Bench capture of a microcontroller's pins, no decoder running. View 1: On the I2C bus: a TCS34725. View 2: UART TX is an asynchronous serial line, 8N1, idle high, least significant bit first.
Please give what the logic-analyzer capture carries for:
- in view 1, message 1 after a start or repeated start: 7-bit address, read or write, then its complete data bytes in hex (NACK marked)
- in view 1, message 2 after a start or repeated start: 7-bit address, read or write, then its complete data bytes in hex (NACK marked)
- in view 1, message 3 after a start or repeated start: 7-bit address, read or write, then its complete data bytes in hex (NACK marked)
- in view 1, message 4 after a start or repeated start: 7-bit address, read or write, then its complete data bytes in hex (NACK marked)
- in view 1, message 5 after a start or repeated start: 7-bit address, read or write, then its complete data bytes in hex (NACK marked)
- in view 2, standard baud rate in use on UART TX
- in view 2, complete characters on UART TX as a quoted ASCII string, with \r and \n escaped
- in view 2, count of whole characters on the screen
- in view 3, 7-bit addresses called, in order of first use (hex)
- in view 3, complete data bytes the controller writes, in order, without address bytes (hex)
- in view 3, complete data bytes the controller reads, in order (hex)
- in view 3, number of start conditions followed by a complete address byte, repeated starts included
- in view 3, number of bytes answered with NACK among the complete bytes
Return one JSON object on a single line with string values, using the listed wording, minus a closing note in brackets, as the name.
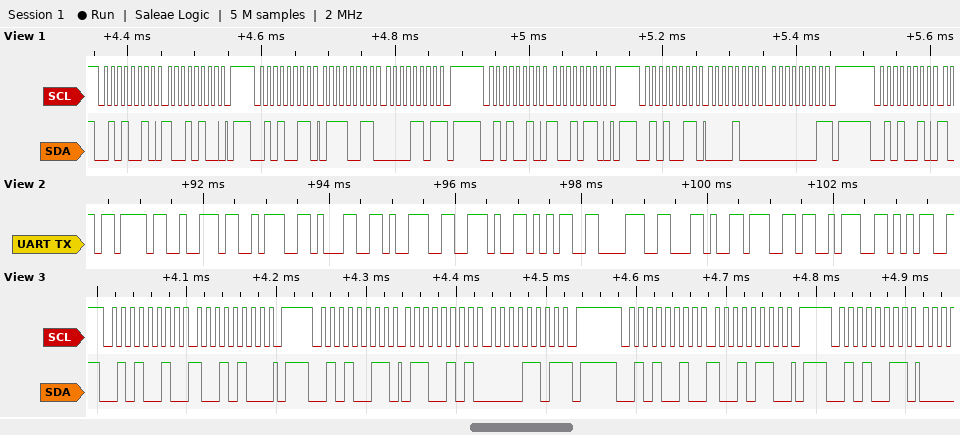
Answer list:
{"in view 1, message 1 after a start or repeated start: 7-bit address, read or write, then its complete data bytes in hex": "0x29 write: 94", "in view 1, message 2 after a start or repeated start: 7-bit address, read or write, then its complete data bytes in hex": "0x29 read: 73 0D NACK", "in view 1, message 3 after a start or repeated start: 7-bit address, read or write, then its complete data bytes in hex": "0x29 write: 96", "in view 1, message 4 after a start or repeated start: 7-bit address, read or write, then its complete data bytes in hex": "0x29 read: 08 01 NACK", "in view 1, message 5 after a start or repeated start: 7-bit address, read or write, then its complete data bytes in hex": "0x29 write", "in view 2, standard baud rate in use on UART TX": "9600 baud", "in view 2, complete characters on UART TX as a quoted ASCII string, with \\r and \\n escaped": "\"{r:19.58,g:5\"", "in view 2, count of whole characters on the screen": "12", "in view 3, 7-bit addresses called, in order of first use": "0x29", "in view 3, complete data bytes the controller writes, in order, without address bytes": "94 96", "in view 3, complete data bytes the controller reads, in order": "65 0D", "in view 3, number of start conditions followed by a complete address byte, repeated starts included": "4", "in view 3, number of bytes answered with NACK among the complete bytes": "1"}
